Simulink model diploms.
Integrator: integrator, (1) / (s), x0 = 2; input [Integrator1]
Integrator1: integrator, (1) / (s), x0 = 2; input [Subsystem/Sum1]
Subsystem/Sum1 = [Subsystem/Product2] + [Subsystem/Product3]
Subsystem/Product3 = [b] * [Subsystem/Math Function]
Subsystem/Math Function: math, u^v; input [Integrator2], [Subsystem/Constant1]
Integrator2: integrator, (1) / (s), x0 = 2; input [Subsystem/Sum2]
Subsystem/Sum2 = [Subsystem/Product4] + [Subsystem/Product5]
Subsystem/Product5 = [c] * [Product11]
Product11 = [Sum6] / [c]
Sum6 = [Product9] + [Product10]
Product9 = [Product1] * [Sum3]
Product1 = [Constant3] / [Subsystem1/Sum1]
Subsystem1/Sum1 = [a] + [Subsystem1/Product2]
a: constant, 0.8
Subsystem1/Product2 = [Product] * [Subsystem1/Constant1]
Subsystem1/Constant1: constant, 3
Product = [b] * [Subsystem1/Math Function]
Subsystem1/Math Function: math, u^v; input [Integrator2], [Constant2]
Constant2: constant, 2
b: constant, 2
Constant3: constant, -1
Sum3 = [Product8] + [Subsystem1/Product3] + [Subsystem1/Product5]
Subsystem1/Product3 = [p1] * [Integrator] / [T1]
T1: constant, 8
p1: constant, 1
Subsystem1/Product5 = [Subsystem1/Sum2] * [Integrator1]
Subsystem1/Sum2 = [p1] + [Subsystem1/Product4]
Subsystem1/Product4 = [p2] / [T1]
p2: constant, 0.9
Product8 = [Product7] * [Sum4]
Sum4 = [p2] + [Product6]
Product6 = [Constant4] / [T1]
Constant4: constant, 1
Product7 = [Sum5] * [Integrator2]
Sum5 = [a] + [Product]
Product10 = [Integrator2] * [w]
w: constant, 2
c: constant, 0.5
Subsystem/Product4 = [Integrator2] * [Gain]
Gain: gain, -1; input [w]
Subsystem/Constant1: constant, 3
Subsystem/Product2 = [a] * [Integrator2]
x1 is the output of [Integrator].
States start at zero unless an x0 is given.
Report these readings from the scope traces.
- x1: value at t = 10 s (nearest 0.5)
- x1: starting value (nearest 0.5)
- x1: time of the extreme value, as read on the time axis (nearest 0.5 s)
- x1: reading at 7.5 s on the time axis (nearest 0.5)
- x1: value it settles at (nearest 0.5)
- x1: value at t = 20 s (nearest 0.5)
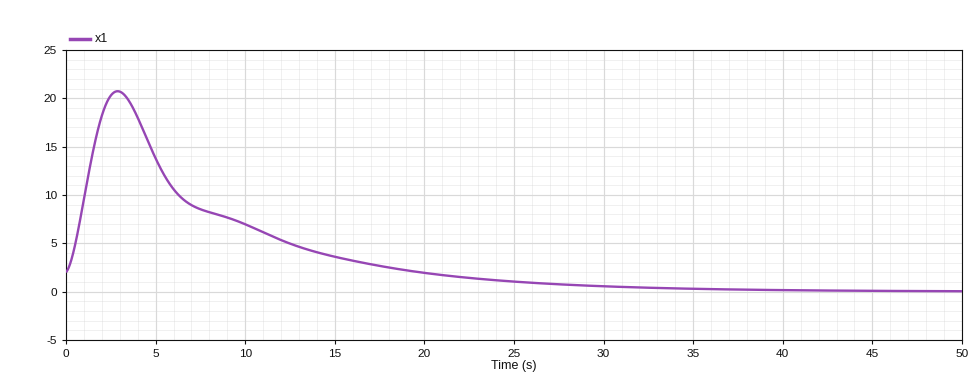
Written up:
7.0
2.0
3.0 s
8.5
0.0
2.0
